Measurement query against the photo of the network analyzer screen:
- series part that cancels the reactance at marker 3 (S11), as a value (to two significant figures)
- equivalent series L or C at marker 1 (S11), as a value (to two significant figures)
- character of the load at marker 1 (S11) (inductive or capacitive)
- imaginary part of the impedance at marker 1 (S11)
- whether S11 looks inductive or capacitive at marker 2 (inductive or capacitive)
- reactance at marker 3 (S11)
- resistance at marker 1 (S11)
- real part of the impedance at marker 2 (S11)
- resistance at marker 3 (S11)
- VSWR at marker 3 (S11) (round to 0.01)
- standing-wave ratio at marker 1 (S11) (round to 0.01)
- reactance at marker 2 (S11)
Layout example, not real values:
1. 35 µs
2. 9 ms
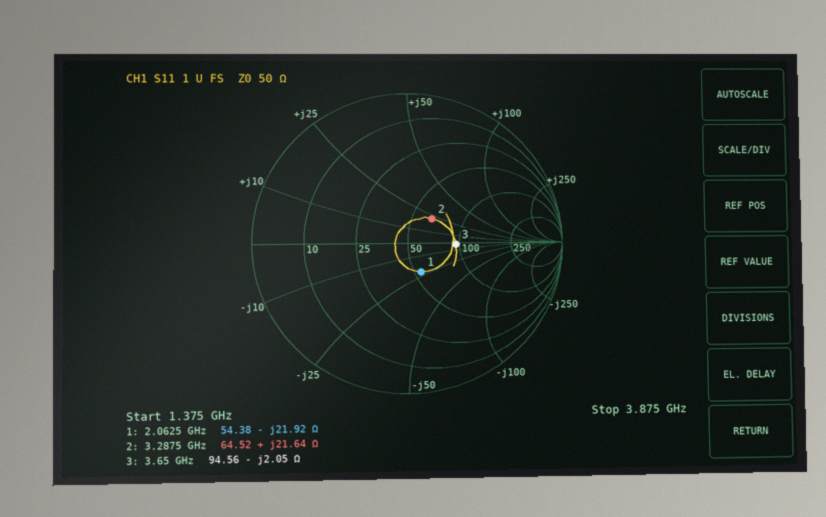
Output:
1. 89 pH
2. 3.5 pF
3. capacitive
4. -21.92 Ω
5. inductive
6. -2.05 Ω
7. 54.38 Ω
8. 64.52 Ω
9. 94.56 Ω
10. 1.89
11. 1.53
12. +21.64 Ω
